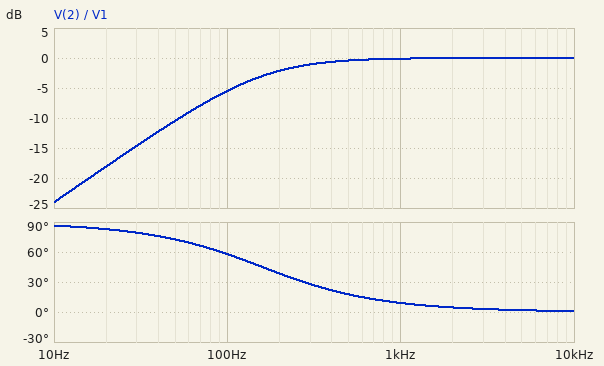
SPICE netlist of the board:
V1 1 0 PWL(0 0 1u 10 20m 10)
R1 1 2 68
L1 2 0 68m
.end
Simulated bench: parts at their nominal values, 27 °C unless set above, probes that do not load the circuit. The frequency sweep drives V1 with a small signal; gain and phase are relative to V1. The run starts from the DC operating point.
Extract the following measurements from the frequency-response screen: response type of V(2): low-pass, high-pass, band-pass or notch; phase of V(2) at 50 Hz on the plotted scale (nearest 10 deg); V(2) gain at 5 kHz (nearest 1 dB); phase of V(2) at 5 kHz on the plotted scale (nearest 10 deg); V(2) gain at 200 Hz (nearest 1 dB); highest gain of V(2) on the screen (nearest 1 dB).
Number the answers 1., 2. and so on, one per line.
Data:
1. high-pass
2. 70 deg
3. 0 dB
4. 0 deg
5. -2 dB
6. 0 dB
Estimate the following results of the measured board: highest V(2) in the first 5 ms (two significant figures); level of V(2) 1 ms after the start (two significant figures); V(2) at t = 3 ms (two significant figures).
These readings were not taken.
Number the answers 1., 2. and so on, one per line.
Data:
1. 10 V
2. 3.7 V
3. 500 mV
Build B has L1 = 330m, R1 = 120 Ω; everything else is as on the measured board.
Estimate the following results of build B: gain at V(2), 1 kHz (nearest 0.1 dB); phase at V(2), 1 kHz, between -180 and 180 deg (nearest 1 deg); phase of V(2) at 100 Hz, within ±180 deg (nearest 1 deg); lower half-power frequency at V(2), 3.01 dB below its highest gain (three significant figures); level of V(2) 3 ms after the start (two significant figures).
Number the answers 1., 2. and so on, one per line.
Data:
1. 0 dB
2. 3 deg
3. 30 deg
4. 57.9 Hz
5. 3.4 V
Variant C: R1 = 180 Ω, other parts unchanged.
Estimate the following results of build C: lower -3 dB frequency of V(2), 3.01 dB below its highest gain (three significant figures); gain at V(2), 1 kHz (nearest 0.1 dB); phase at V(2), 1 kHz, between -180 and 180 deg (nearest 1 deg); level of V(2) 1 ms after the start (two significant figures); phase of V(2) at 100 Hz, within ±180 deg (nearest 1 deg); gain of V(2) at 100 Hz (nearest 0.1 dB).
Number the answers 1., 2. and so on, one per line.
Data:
1. 421 Hz
2. -0.7 dB
3. 23 deg
4. 710 mV
5. 77 deg
6. -12.7 dB
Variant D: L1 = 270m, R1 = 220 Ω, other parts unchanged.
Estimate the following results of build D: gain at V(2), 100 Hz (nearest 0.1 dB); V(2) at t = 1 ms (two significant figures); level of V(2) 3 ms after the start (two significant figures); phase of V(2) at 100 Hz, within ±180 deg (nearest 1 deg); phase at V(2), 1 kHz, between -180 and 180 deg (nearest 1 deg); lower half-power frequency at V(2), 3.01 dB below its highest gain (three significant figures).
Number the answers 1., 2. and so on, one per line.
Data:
1. -4.3 dB
2. 4.4 V
3. 870 mV
4. 52 deg
5. 7 deg
6. 130 Hz
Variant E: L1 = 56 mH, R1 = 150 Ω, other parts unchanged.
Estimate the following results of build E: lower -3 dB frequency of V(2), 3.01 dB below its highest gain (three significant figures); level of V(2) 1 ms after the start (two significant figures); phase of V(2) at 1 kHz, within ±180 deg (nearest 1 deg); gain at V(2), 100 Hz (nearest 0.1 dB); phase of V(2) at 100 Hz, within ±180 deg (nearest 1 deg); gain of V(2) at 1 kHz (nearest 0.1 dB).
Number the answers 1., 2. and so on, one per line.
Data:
1. 426 Hz
2. 690 mV
3. 23 deg
4. -12.8 dB
5. 77 deg
6. -0.7 dB
